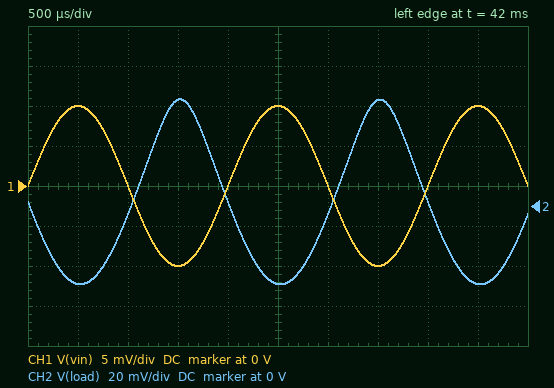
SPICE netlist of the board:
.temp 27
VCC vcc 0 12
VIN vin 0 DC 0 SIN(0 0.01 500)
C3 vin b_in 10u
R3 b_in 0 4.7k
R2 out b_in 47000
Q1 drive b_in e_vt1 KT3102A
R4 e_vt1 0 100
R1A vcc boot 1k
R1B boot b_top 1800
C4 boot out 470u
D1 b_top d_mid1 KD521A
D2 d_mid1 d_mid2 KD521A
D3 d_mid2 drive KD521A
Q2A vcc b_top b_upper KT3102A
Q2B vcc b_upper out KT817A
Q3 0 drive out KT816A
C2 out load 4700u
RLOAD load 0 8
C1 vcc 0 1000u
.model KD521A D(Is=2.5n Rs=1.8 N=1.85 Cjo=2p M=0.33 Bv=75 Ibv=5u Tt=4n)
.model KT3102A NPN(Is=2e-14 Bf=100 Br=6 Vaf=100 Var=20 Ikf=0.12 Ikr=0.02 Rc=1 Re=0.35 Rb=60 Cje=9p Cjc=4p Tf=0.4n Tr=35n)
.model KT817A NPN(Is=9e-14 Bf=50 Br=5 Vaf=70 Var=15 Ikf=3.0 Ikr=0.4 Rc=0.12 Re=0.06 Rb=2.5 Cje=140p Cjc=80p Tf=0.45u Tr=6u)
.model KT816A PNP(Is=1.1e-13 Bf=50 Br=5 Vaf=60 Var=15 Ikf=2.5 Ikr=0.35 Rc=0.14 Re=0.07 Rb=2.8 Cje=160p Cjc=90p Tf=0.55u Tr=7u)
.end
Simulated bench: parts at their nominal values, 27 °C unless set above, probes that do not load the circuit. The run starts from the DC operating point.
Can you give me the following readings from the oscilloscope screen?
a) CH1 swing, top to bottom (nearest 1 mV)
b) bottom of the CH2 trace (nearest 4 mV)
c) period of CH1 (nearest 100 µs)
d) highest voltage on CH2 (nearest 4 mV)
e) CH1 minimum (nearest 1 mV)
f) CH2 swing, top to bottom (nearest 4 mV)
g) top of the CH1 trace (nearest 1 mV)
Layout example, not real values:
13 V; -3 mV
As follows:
20 mV; -40 mV; 2.0 ms; 52 mV; -10 mV; 92 mV; 10 mV
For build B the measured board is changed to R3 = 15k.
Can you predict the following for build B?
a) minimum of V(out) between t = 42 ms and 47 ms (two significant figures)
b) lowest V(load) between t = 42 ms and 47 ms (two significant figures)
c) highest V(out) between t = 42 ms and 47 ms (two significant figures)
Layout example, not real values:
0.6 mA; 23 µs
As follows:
4.9 V; -50 mV; 5.0 V
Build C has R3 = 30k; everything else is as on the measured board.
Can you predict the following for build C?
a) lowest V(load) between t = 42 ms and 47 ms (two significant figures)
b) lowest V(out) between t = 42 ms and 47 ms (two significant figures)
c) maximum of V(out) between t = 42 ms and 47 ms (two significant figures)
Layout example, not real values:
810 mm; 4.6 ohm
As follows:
-51 mV; 3.9 V; 4.0 V
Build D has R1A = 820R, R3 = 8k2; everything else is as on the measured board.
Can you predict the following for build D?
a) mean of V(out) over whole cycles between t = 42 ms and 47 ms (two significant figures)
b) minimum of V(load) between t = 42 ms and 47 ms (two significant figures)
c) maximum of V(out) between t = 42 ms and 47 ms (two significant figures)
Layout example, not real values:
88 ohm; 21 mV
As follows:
6.5 V; -48 mV; 6.6 V
